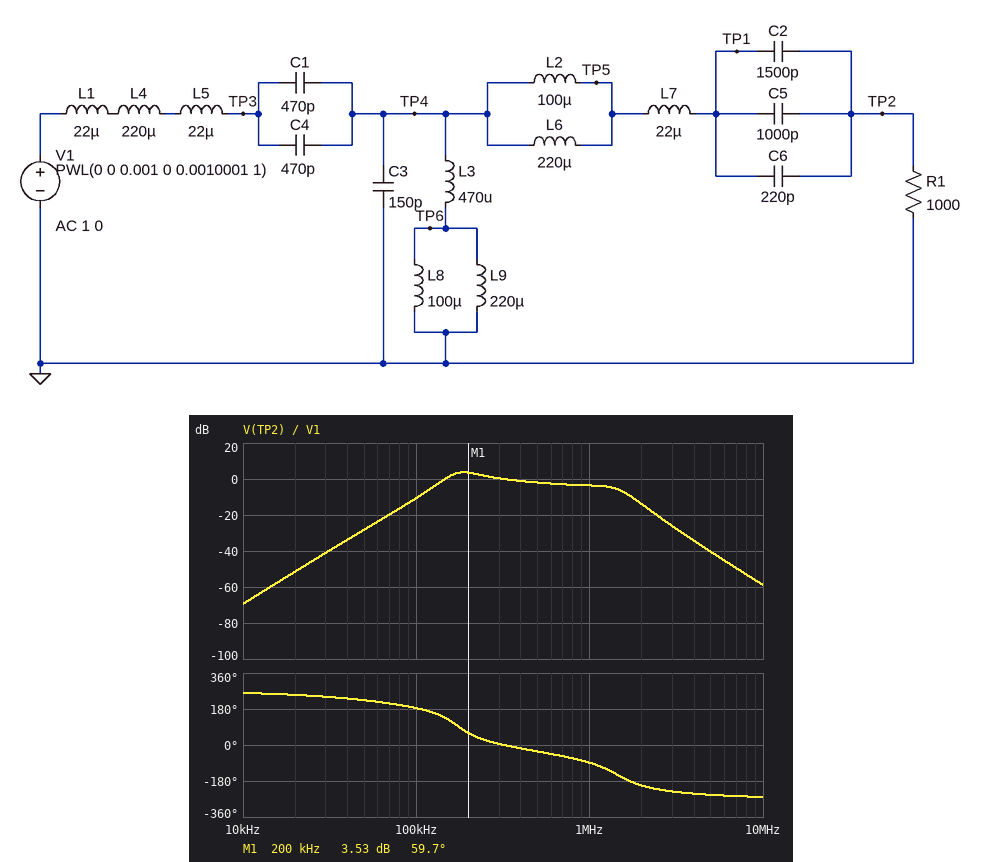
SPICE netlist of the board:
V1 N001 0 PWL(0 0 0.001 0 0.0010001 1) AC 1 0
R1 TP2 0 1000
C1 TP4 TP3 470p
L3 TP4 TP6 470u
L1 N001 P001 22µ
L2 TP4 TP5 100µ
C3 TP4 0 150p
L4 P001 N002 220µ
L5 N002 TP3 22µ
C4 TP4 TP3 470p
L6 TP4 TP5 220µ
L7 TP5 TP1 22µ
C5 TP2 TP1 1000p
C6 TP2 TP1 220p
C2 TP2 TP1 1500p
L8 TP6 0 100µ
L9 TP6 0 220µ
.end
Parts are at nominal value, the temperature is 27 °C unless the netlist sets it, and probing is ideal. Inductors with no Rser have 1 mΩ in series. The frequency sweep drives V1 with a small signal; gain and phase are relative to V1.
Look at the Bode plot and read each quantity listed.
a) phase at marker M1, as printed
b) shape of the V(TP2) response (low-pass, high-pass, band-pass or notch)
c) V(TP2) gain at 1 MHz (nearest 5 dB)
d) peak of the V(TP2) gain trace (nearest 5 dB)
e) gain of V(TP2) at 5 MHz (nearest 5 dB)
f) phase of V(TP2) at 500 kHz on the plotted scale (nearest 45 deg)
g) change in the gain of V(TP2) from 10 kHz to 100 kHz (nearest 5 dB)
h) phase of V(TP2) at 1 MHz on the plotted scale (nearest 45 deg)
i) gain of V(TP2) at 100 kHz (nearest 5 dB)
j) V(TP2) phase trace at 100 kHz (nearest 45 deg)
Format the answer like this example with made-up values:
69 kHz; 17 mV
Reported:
59.7 deg; band-pass; -5 dB; 5 dB; -40 dB; -45 deg; 60 dB; -90 deg; -10 dB; 180 deg
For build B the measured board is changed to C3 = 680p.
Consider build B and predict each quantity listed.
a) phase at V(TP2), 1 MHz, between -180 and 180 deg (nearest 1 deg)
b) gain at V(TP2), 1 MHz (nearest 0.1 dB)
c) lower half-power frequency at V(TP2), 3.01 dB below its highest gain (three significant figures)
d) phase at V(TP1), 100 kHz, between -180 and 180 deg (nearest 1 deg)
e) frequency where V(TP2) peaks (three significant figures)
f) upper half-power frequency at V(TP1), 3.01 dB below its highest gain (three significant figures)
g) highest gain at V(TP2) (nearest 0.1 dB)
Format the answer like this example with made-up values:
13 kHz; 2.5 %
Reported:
168 deg; -14.0 dB; 408 kHz; 149 deg; 523 kHz; 608 kHz; 4.9 dB
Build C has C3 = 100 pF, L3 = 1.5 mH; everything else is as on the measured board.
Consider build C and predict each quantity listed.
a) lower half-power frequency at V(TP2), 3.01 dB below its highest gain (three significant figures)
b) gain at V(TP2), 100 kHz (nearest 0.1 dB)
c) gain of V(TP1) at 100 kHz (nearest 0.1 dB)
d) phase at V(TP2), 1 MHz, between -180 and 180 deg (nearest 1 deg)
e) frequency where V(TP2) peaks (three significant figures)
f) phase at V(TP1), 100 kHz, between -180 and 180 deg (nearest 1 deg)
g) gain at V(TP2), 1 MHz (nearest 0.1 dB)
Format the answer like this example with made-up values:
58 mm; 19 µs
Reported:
96.3 kHz; -2.7 dB; -1.4 dB; -82 deg; 280 kHz; 79 deg; -4.2 dB
